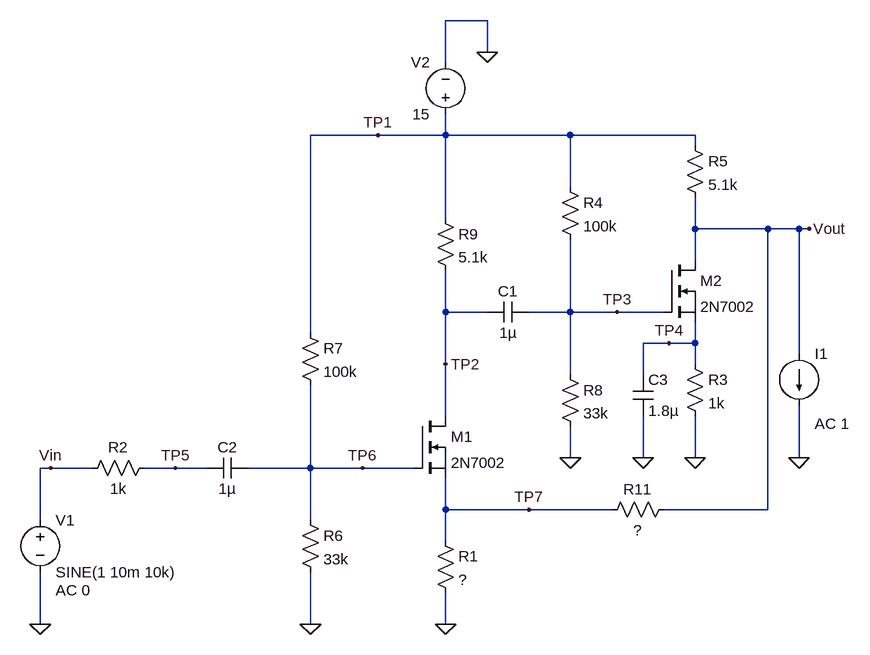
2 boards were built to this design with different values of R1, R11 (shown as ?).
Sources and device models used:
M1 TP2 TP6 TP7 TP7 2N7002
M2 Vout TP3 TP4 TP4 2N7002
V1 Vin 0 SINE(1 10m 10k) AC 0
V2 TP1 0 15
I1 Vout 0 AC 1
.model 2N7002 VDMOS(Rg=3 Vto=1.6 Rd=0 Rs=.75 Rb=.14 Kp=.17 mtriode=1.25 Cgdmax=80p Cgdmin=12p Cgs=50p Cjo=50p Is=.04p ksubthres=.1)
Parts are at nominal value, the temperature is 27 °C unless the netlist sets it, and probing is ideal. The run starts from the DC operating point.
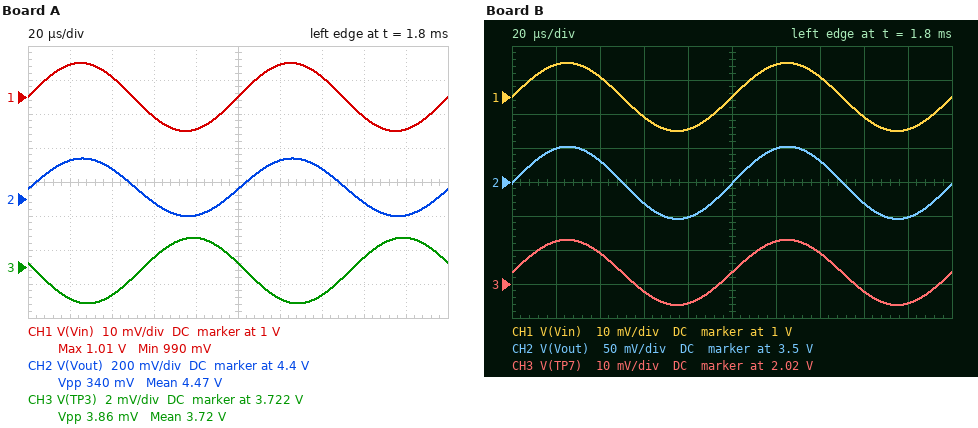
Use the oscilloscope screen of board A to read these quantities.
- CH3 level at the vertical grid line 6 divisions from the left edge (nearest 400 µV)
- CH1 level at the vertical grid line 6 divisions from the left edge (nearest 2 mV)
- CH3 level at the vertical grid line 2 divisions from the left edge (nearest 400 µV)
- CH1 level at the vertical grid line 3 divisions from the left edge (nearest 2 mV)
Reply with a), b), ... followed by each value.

a) 3.7200 V
b) 1.010 V
c) 3.7204 V
d) 994 mV
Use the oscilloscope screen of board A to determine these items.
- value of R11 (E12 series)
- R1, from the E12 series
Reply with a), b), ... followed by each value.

a) 33 kΩ
b) 1.8 kΩ
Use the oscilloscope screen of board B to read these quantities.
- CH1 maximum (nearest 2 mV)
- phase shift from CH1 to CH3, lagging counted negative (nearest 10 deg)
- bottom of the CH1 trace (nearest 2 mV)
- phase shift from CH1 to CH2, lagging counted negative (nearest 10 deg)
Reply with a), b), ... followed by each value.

a) 1.010 V
b) 0 deg
c) 990 mV
d) 0 deg
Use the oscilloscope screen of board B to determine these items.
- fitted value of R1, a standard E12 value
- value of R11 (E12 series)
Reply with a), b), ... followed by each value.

a) 1.2 kΩ
b) 5.6 kΩ
